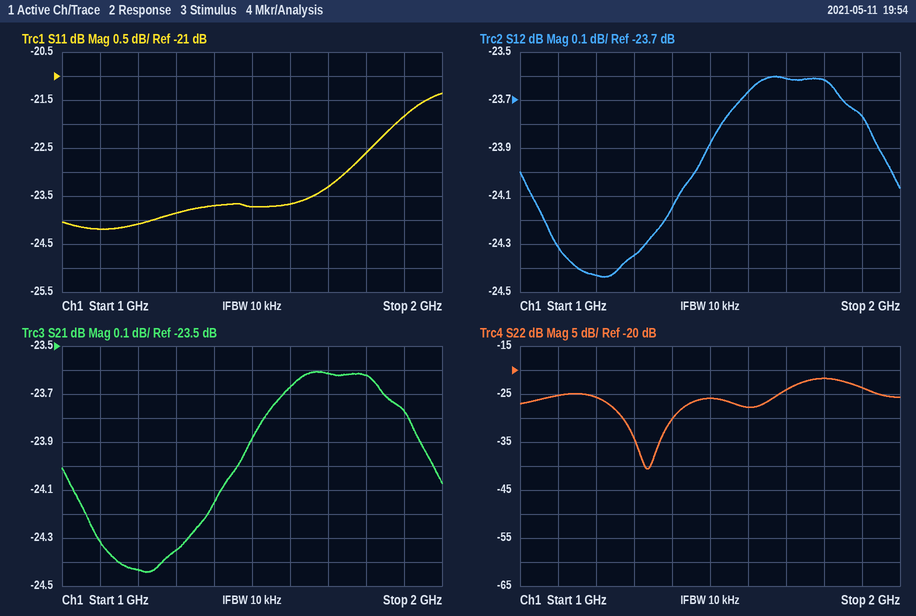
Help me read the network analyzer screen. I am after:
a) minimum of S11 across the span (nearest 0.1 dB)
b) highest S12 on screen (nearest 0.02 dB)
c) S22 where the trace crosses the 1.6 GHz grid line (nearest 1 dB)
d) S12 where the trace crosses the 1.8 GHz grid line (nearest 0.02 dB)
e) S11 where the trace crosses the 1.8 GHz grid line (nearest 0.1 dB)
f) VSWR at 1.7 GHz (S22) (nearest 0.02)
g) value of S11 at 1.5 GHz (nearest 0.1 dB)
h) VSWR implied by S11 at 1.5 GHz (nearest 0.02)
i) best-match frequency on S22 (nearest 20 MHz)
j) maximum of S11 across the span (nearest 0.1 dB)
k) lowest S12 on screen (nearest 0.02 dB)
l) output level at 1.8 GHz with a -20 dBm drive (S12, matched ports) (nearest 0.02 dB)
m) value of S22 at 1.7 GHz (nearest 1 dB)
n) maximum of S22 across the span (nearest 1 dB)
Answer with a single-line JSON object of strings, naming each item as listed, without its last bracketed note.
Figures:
{"minimum of S11 across the span": "-24.2 dB", "highest S12 on screen": "-23.60 dB", "S22 where the trace crosses the 1.6 GHz grid line": "-28 dB", "S12 where the trace crosses the 1.8 GHz grid line": "-23.62 dB", "S11 where the trace crosses the 1.8 GHz grid line": "-22.6 dB", "VSWR at 1.7 GHz (S22)": "1.14", "value of S11 at 1.5 GHz": "-23.7 dB", "VSWR implied by S11 at 1.5 GHz": "1.14", "best-match frequency on S22": "1.34 GHz", "maximum of S11 across the span": "-21.4 dB", "lowest S12 on screen": "-24.44 dB", "output level at 1.8 GHz with a -20 dBm drive (S12, matched ports)": "-43.62 dBm", "value of S22 at 1.7 GHz": "-24 dB", "maximum of S22 across the span": "-22 dB"}
